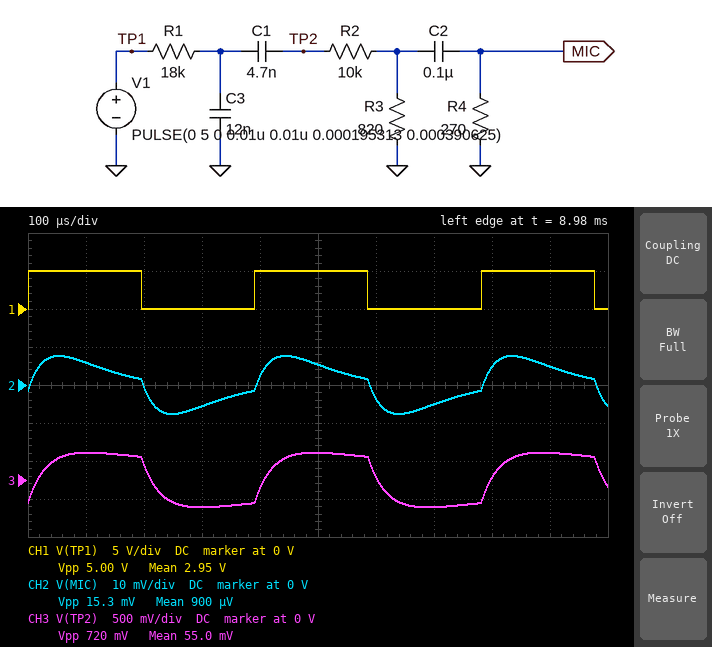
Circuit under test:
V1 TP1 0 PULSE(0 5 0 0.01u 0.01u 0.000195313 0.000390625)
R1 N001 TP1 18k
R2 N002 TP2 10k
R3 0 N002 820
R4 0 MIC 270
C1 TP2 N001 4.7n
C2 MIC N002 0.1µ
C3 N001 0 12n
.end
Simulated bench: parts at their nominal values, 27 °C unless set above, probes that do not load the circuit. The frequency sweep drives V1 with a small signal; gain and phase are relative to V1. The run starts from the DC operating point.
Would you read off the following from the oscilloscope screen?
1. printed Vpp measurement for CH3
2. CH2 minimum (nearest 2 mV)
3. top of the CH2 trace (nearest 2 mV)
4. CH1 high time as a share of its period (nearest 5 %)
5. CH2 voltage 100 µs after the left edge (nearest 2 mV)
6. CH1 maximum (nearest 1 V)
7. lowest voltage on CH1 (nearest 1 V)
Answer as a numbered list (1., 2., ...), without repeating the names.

1. 720 mV
2. -8 mV
3. 8 mV
4. 50 %
5. 6 mV
6. 5 V
7. 0 V
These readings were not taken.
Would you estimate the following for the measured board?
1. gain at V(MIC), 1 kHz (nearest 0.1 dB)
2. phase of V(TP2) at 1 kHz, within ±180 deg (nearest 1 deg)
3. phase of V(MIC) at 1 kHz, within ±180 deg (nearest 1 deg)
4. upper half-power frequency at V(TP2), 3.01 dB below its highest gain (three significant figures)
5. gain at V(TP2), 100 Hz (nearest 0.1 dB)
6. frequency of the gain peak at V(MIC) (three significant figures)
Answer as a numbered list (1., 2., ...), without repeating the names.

1. -56.6 dB
2. 13 deg
3. 70 deg
4. 5.55 kHz
5. -30.1 dB
6. 2.79 kHz
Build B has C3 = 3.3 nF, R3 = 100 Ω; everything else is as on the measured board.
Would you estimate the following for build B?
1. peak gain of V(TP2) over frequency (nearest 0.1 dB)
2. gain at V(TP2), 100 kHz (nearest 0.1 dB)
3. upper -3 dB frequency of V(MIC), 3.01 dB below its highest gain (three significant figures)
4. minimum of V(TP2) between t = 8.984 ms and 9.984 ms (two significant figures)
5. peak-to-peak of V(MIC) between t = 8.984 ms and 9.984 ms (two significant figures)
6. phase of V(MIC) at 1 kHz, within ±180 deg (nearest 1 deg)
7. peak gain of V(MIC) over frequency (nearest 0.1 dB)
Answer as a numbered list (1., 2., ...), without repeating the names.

1. -12.1 dB
2. -31.5 dB
3. 17.0 kHz
4. -780 mV
5. 11 mV
6. 113 deg
7. -57.4 dB
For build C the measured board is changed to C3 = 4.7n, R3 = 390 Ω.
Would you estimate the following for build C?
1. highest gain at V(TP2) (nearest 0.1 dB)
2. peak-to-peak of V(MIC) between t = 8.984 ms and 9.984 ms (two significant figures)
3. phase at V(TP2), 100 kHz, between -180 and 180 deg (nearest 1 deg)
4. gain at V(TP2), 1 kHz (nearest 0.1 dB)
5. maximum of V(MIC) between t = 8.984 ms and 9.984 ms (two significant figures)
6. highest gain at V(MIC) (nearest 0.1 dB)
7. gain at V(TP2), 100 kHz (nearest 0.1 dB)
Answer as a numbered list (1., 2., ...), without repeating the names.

1. -13.1 dB
2. 22 mV
3. -85 deg
4. -14.4 dB
5. 11 mV
6. -50.9 dB
7. -34.5 dB
